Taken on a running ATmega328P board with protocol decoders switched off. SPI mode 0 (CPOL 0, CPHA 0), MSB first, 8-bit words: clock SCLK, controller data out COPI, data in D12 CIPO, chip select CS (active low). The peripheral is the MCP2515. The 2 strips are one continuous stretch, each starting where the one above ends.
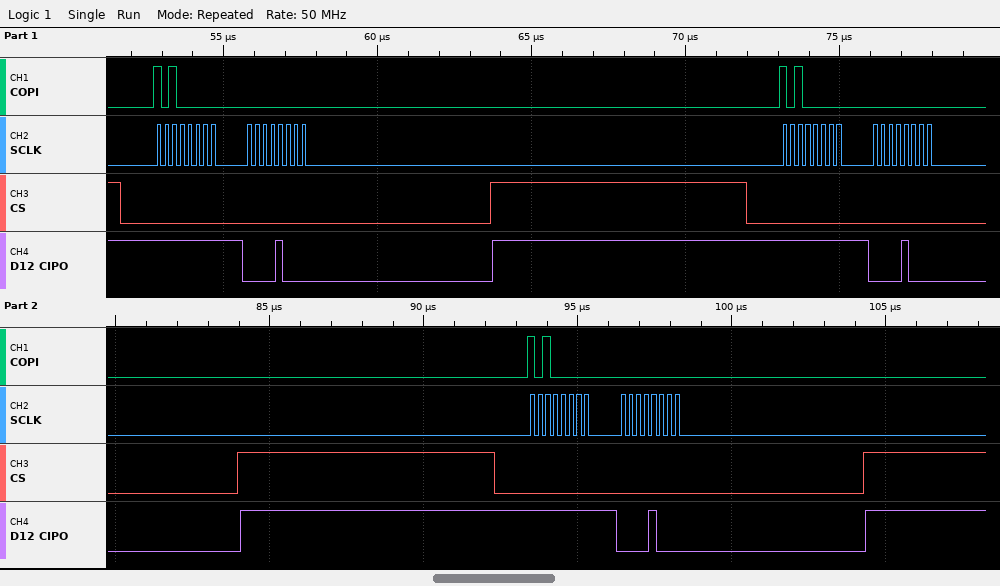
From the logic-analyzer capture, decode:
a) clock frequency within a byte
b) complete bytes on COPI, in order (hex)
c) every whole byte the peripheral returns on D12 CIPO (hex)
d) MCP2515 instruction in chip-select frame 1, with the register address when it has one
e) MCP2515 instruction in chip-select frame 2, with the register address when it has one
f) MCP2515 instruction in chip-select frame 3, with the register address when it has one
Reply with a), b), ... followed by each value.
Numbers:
a) 4 MHz
b) A0 00 A0 00 A0 00
c) FF 08 FF 08 FF 08
d) READ STATUS
e) READ STATUS
f) READ STATUS
